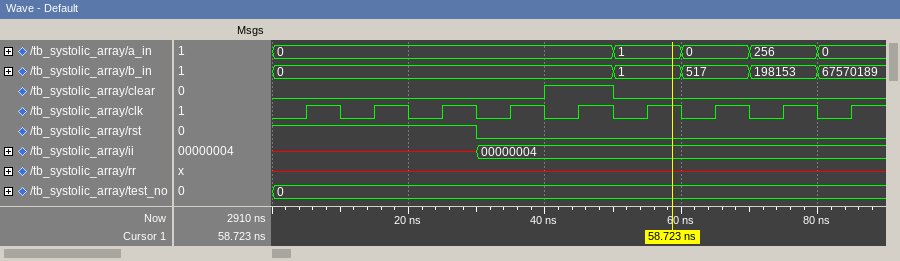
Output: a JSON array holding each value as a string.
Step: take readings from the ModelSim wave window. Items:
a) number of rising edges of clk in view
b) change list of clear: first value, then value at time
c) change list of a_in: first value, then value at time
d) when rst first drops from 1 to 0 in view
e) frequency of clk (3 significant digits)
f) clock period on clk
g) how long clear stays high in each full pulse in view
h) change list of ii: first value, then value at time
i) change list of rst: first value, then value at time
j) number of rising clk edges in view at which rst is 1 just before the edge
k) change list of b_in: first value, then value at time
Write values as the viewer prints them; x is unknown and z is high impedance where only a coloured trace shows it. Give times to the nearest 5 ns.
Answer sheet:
["9", "0, 1 at 40 ns, 0 at 50 ns", "0, 1 at 50 ns, 0 at 60 ns, 256 at 70 ns, 0 at 80 ns", "30 ns", "100 MHz", "10 ns", "10 ns", "x, 00000004 at 30 ns", "1, 0 at 30 ns", "3", "0, 1 at 50 ns, 517 at 60 ns, 198153 at 70 ns, 67570189 at 80 ns"]
